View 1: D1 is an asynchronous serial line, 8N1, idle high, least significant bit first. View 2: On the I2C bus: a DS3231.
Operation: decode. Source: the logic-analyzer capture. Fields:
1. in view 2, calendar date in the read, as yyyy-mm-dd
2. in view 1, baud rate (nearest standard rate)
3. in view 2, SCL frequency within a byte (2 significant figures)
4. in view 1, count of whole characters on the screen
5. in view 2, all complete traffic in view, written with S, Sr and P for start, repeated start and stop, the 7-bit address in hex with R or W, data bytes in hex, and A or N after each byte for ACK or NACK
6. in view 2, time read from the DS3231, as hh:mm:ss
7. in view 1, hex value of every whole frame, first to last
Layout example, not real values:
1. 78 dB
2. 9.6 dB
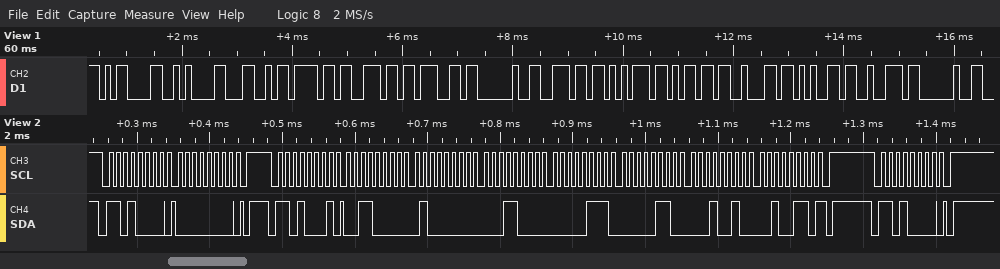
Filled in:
1. 2026-12-06
2. 9600 baud
3. 100 kHz
4. 14
5. S 68W A 00 A P S 68R A 30 A 40 A 18 A 07 A 06 A 12 A 26 N P S 68W A P
6. 18:40:30
7. 0x0D 0x0A 0x4C 0x6F 0x6E 0x67 0x20 0x6E 0x75 0x6D 0x62 0x65 0x72 0x20
